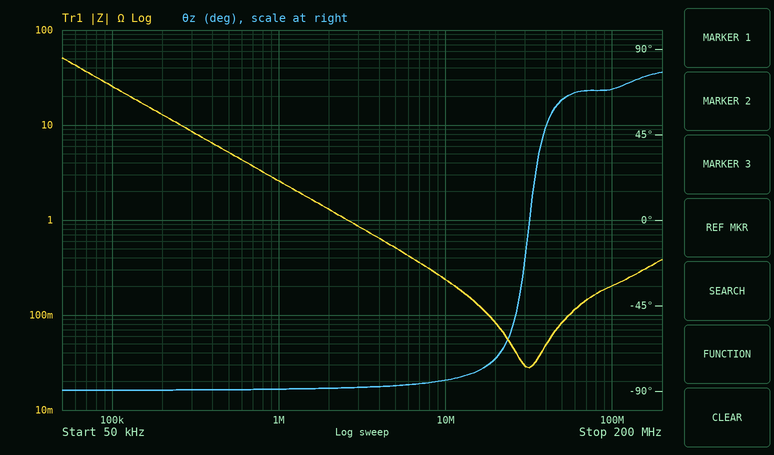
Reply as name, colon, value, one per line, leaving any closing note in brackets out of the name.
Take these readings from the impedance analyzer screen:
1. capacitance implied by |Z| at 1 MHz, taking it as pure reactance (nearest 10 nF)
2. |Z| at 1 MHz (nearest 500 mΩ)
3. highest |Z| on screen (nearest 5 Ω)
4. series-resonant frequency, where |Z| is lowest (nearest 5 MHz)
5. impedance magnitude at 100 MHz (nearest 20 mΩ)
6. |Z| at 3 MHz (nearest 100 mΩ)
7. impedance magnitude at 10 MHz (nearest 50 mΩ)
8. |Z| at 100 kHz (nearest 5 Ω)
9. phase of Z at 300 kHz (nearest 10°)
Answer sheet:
capacitance implied by |Z| at 1 MHz, taking it as pure reactance: 60 nF
|Z| at 1 MHz: 2.5 Ω
highest |Z| on screen: 50 Ω
series-resonant frequency, where |Z| is lowest: 30 MHz
impedance magnitude at 100 MHz: 200 mΩ
|Z| at 3 MHz: 900 mΩ
impedance magnitude at 10 MHz: 250 mΩ
|Z| at 100 kHz: 25 Ω
phase of Z at 300 kHz: -90°
